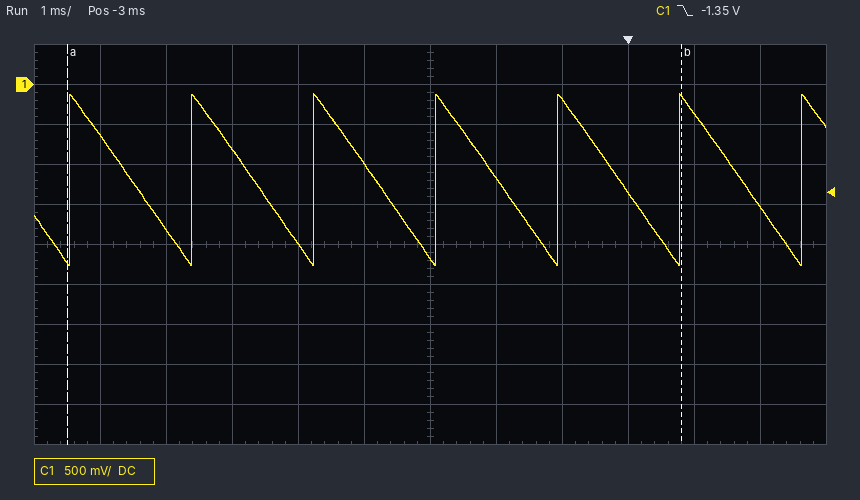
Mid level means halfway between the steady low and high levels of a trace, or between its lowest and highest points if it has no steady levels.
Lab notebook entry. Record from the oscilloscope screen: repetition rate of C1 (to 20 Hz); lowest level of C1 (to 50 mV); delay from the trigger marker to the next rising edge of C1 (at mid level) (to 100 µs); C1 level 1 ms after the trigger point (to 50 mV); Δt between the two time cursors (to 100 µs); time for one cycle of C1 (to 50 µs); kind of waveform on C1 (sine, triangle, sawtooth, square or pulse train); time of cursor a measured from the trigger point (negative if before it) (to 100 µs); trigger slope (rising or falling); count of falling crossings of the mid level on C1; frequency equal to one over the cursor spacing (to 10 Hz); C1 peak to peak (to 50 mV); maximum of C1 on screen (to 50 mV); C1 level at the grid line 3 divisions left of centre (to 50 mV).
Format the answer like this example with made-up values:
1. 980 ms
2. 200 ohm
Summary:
1. 540 Hz
2. -2.25 V
3. 800 µs
4. -350 mV
5. 9.3 ms
6. 1.85 ms
7. sawtooth
8. -8.5 ms
9. falling
10. 6
11. 110 Hz
12. 2.15 V
13. -100 mV
14. -800 mV
